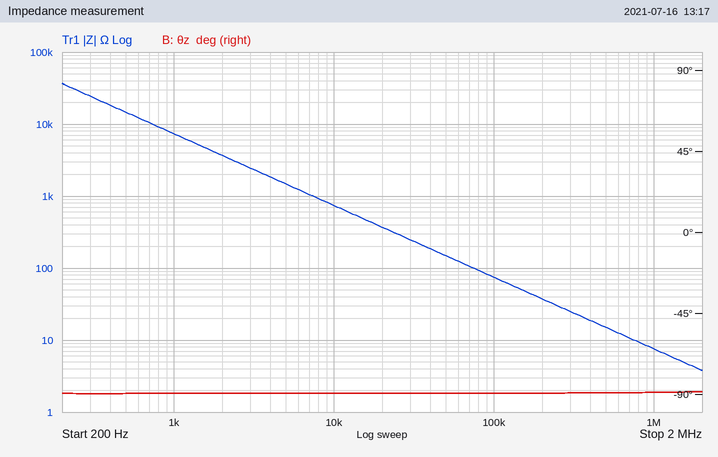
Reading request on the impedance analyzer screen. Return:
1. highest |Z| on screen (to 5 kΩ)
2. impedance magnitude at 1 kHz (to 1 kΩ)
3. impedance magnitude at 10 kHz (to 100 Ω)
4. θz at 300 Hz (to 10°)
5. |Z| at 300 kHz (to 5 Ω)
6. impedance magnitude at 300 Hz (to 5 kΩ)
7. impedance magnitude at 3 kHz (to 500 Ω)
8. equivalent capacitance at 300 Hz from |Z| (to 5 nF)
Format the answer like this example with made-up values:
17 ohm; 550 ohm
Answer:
35 kΩ; 7 kΩ; 700 Ω; -90°; 25 Ω; 25 kΩ; 2.5 kΩ; 20 nF
